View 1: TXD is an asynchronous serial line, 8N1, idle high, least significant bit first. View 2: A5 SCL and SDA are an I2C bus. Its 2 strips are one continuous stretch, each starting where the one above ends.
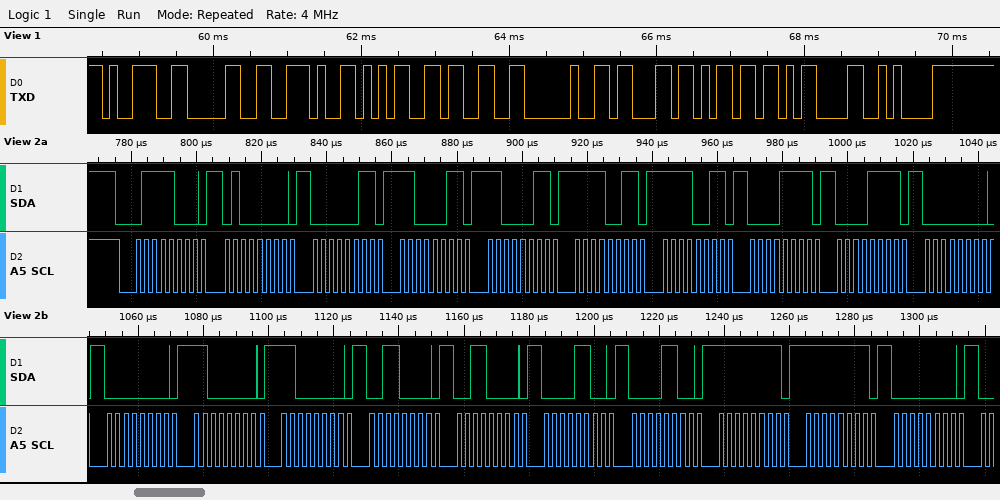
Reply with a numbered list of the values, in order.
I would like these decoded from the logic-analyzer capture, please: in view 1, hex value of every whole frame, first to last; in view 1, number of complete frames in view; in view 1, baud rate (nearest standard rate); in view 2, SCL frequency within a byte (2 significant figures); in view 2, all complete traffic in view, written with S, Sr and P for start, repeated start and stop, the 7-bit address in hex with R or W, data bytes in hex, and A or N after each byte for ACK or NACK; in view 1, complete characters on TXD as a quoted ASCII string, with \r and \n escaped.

1. 39 30 2E 35 33 20 63 6D 0D 0A
2. 10
3. 9600 baud
4. 400 kHz
5. S 3CW A 40 A 03 A C3 A C3 A F3 A F3 A 0F A 0F A 00 A 00 A C0 A C0 A 30 A 30 A 0C A 0C A FF A FF A 00 A
6. "90.53 cm\r\n"
